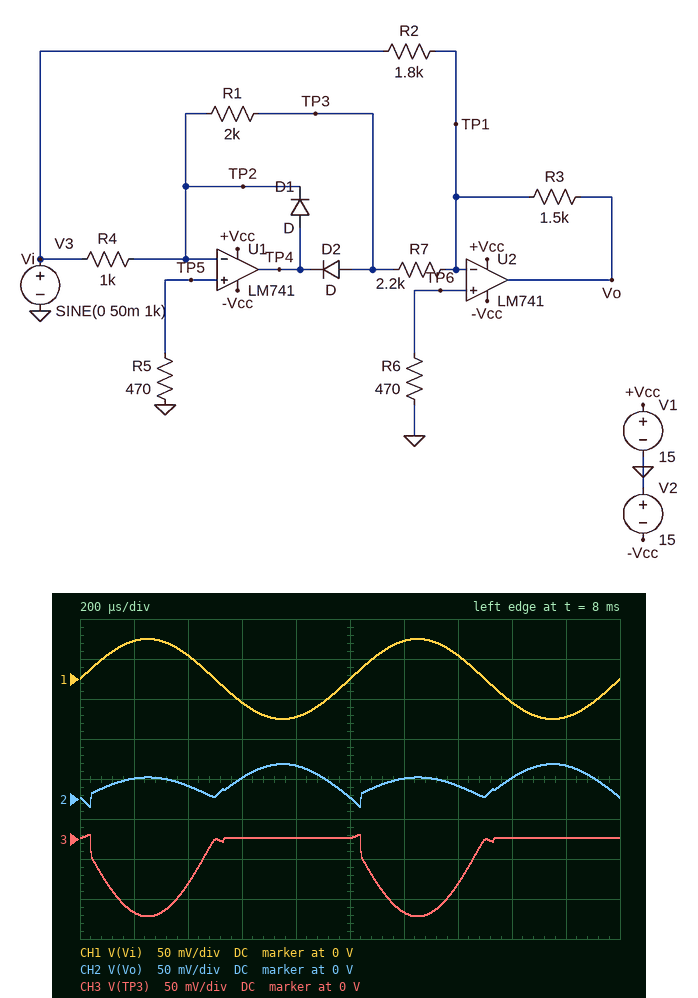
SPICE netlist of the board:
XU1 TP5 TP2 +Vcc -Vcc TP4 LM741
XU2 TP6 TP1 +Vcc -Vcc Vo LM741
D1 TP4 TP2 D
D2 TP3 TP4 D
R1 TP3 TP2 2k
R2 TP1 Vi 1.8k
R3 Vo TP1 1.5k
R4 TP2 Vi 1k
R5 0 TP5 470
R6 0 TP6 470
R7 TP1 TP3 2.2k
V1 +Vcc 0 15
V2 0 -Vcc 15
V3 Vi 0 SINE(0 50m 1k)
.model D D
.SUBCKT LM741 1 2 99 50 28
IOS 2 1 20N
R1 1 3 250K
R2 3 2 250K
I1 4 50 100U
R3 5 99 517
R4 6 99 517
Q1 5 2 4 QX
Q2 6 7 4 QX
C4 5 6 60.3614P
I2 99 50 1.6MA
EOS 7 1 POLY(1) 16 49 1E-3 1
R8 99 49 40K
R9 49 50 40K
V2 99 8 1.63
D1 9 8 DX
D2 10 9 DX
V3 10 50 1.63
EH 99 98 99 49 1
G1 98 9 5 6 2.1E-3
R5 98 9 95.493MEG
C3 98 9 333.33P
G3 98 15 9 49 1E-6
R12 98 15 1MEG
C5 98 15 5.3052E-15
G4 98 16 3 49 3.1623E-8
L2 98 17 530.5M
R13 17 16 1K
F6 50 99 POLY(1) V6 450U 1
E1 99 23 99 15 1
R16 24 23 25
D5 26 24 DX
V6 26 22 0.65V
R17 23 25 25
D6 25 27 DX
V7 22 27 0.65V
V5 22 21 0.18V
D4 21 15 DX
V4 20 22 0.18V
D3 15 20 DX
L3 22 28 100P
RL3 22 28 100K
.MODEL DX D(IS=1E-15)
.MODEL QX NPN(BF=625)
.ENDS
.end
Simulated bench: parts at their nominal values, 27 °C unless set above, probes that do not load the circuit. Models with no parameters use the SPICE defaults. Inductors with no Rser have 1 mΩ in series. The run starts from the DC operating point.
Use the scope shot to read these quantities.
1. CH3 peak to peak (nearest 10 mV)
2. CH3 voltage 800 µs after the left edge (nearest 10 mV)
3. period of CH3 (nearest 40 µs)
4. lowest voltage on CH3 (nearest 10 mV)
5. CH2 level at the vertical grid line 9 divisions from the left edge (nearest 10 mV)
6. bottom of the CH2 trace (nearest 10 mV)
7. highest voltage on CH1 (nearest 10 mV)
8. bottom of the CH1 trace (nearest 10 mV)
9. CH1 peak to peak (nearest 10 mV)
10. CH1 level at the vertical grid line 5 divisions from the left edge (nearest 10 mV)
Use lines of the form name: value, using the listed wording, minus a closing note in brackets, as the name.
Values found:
CH3 peak to peak: 100 mV
CH3 voltage 800 µs after the left edge: 0 V
period of CH3: 1.00 ms
lowest voltage on CH3: -100 mV
CH2 level at the vertical grid line 9 divisions from the left edge: 40 mV
bottom of the CH2 trace: -10 mV
highest voltage on CH1: 50 mV
bottom of the CH1 trace: -50 mV
CH1 peak to peak: 100 mV
CH1 level at the vertical grid line 5 divisions from the left edge: 0 V
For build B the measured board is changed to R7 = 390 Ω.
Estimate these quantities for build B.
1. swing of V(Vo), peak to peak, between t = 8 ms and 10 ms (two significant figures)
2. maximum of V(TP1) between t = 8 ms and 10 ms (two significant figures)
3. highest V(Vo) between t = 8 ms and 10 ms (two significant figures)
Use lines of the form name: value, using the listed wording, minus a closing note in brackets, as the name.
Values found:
swing of V(Vo), peak to peak, between t = 8 ms and 10 ms: 350 mV
maximum of V(TP1) between t = 8 ms and 10 ms: 1.3 mV
highest V(Vo) between t = 8 ms and 10 ms: 340 mV
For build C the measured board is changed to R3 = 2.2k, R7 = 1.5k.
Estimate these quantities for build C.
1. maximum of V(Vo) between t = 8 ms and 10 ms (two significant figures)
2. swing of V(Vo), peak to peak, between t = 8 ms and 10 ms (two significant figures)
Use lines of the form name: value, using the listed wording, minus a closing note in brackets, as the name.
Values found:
maximum of V(Vo) between t = 8 ms and 10 ms: 85 mV
swing of V(Vo), peak to peak, between t = 8 ms and 10 ms: 100 mV
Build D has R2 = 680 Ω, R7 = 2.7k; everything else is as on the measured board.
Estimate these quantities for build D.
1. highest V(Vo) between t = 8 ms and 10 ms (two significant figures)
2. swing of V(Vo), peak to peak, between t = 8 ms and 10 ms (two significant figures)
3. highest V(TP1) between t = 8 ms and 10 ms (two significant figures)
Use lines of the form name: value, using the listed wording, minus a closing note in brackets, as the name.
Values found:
highest V(Vo) between t = 8 ms and 10 ms: 110 mV
swing of V(Vo), peak to peak, between t = 8 ms and 10 ms: 170 mV
highest V(TP1) between t = 8 ms and 10 ms: 1.1 mV
